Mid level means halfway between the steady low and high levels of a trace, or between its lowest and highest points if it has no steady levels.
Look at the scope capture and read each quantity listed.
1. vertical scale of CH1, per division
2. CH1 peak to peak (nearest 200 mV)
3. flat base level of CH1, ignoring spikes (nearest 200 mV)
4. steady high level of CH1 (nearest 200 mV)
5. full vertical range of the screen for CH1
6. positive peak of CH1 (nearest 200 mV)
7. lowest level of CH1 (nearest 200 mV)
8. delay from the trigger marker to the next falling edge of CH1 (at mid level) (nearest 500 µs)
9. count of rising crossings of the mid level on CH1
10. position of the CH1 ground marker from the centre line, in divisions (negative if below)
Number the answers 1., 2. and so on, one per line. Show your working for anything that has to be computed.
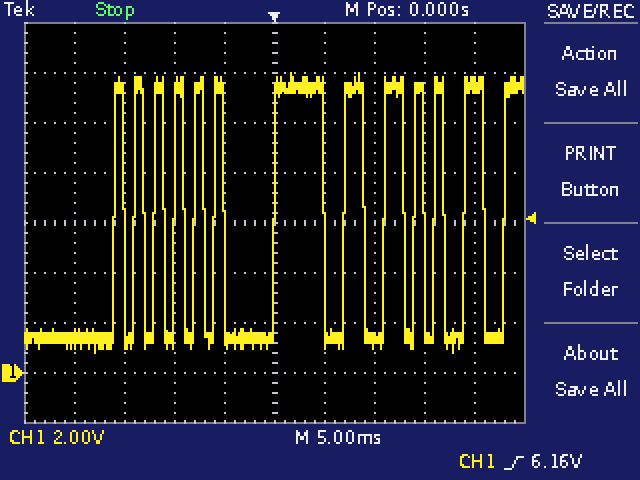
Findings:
1. 2 V
2. 12.0 V − (800 mV) = 11.2 V
3. 1.4 V
4. 11.4 V
5. 16 V
6. 12.0 V
7. 800 mV
8. 5.0 ms
9. 13
10. -3.0 div
